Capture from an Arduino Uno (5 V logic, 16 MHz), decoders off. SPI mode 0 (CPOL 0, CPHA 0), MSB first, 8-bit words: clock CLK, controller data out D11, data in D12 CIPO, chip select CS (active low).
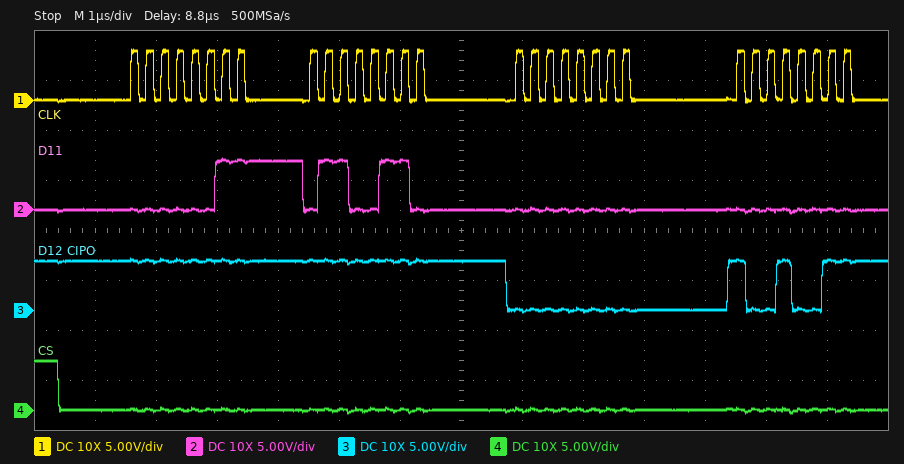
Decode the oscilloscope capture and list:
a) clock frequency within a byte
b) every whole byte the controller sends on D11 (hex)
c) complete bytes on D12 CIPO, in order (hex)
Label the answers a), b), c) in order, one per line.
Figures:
a) 4 MHz
b) 0x03 0x66 0x00 0x00
c) 0xFF 0xFF 0x00 0x93
